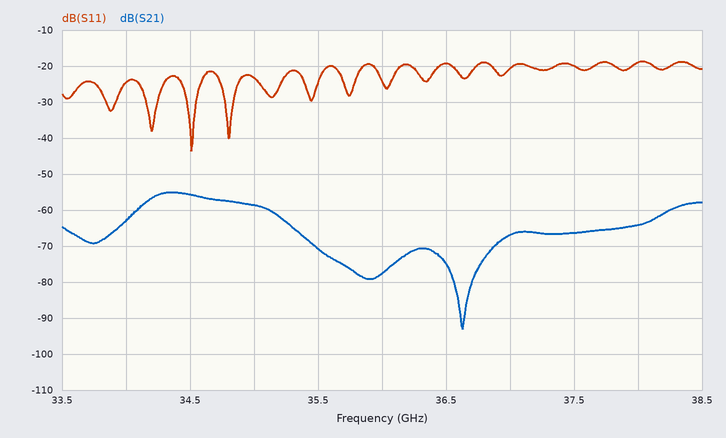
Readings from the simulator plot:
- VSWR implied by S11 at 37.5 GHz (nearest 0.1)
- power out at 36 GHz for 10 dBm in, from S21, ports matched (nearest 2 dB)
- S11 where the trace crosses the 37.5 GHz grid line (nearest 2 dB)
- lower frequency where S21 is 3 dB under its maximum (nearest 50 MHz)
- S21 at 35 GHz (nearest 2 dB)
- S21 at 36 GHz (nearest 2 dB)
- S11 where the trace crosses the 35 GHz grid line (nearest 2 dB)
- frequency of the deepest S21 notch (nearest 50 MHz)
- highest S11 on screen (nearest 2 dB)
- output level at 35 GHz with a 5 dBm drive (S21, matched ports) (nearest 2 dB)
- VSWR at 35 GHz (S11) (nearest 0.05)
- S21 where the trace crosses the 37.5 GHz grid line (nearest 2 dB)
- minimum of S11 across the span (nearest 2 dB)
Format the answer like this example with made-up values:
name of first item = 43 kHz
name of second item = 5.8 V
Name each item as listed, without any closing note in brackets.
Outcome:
VSWR implied by S11 at 37.5 GHz = 1.2
power out at 36 GHz for 10 dBm in, from S21, ports matched = -68 dBm
S11 where the trace crosses the 37.5 GHz grid line = -20 dB
lower frequency where S21 is 3 dB under its maximum = 34.15 GHz
S21 at 35 GHz = -58 dB
S21 at 36 GHz = -78 dB
S11 where the trace crosses the 35 GHz grid line = -24 dB
frequency of the deepest S21 notch = 36.65 GHz
highest S11 on screen = -18 dB
output level at 35 GHz with a 5 dBm drive (S21, matched ports) = -54 dBm
VSWR at 35 GHz (S11) = 1.15
S21 where the trace crosses the 37.5 GHz grid line = -66 dB
minimum of S11 across the span = -44 dB
